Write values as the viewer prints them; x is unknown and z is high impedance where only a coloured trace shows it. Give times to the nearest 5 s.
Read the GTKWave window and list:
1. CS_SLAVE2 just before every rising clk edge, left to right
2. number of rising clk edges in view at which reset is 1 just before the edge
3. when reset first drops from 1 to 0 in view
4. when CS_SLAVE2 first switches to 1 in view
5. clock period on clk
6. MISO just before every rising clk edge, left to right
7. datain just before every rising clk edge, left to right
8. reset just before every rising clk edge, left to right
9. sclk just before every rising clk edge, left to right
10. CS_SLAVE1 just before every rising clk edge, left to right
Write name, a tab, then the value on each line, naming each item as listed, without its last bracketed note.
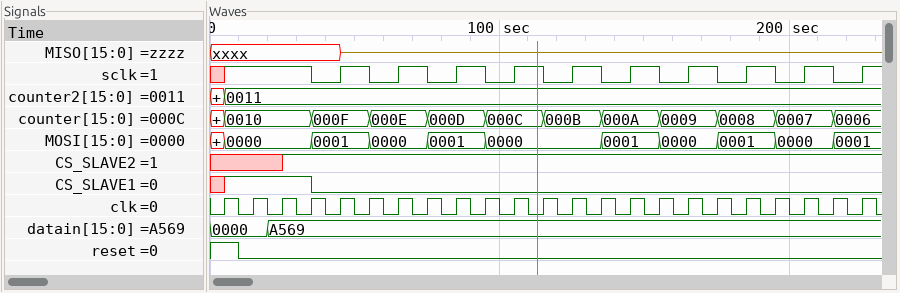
CS_SLAVE2 just before every rising clk edge, left to right	x x x 1 1 1 1 1 1 1 1 1 1 1 1 1 1 1 1 1 1 1 1
number of rising clk edges in view at which reset is 1 just before the edge	1
when reset first drops from 1 to 0 in view	10 s
when CS_SLAVE2 first switches to 1 in view	25 s
clock period on clk	10 s
MISO just before every rising clk edge, left to right	xxxx, xxxx, xxxx, xxxx, xxxx, z, z, z, z, z, z, z, z, z, z, z, z, z, z, z, z, z, z
datain just before every rising clk edge, left to right	0000, 0000, A569, A569, A569, A569, A569, A569, A569, A569, A569, A569, A569, A569, A569, A569, A569, A569, A569, A569, A569, A569, A569
reset just before every rising clk edge, left to right	1 0 0 0 0 0 0 0 0 0 0 0 0 0 0 0 0 0 0 0 0 0 0
sclk just before every rising clk edge, left to right	x 1 1 1 0 1 0 1 0 1 0 1 0 1 0 1 0 1 0 1 0 1 0
CS_SLAVE1 just before every rising clk edge, left to right	x 1 1 1 0 0 0 0 0 0 0 0 0 0 0 0 0 0 0 0 0 0 0
